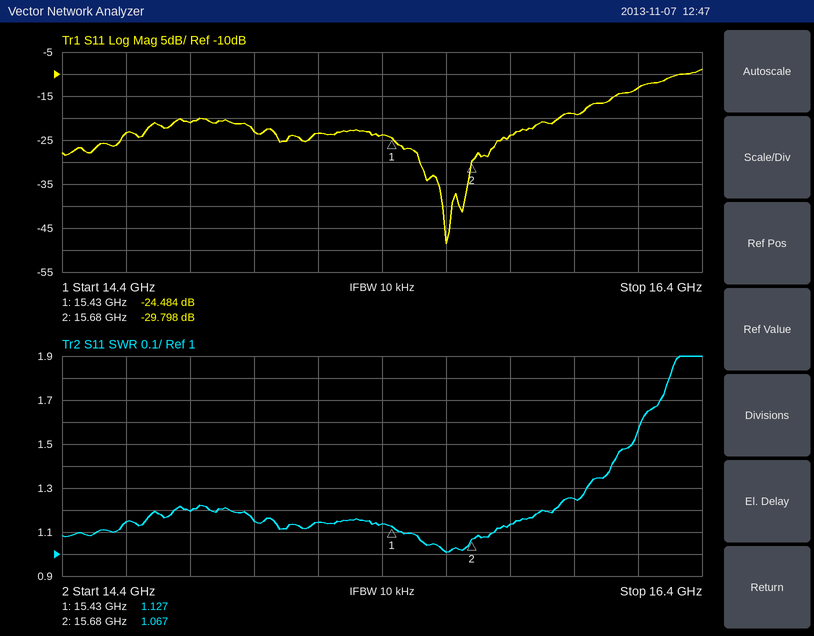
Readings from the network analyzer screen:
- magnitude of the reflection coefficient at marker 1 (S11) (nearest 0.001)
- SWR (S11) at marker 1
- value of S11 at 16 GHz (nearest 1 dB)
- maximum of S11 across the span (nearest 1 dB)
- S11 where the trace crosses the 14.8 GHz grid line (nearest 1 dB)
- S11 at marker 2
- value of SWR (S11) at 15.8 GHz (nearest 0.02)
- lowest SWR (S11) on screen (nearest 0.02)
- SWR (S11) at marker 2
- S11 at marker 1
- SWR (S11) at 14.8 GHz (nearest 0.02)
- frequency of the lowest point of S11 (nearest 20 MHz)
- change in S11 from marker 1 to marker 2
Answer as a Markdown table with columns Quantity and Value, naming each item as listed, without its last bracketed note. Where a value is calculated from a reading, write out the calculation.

| Quantity | Value |
|---|---|
| magnitude of the reflection coefficient at marker 1 (S11) | 10^(-24.484/20) ≈ 0.060 |
| SWR (S11) at marker 1 | 1.127 |
| value of S11 at 16 GHz | -19 dB |
| maximum of S11 across the span | -9 dB |
| S11 where the trace crosses the 14.8 GHz grid line | -21 dB |
| S11 at marker 2 | -29.798 dB |
| value of SWR (S11) at 15.8 GHz | 1.14 |
| lowest SWR (S11) on screen | 1.00 |
| SWR (S11) at marker 2 | 1.067 |
| S11 at marker 1 | -24.484 dB |
| SWR (S11) at 14.8 GHz | 1.20 |
| frequency of the lowest point of S11 | 15.60 GHz |
| change in S11 from marker 1 to marker 2 | -29.798 − (-24.484) = -5.314 dB |
